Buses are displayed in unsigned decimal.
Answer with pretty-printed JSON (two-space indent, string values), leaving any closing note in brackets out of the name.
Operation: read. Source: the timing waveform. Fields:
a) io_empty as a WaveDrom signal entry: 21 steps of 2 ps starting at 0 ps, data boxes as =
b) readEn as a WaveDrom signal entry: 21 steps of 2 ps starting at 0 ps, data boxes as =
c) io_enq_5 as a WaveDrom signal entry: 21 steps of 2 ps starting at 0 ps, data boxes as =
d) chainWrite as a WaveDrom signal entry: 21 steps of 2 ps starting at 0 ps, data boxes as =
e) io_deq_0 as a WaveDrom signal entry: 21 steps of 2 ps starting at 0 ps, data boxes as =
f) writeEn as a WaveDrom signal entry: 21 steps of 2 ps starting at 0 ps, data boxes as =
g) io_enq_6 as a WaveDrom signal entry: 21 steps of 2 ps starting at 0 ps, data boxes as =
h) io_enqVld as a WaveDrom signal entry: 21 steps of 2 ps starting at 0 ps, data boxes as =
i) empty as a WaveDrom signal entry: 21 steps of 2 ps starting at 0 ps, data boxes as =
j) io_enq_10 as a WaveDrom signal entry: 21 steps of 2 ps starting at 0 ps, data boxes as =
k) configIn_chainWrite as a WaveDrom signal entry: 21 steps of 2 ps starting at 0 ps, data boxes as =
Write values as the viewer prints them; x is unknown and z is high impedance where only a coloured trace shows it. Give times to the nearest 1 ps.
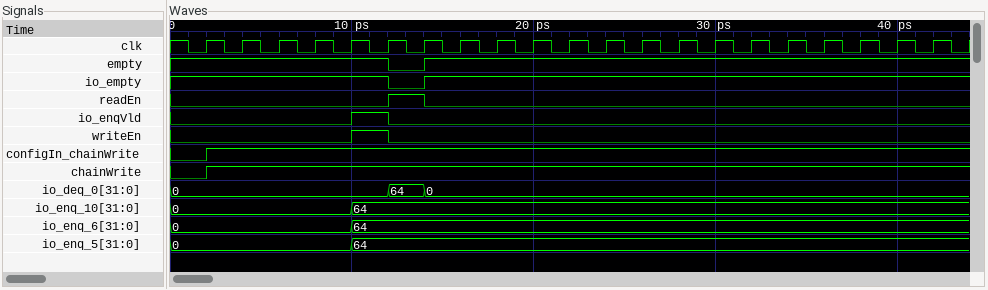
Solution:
{
  "io_empty as a WaveDrom signal entry: 21 steps of 2 ps starting at 0 ps, data boxes as =": "{name: 'io_empty', wave: '1.....01.............'}",
  "readEn as a WaveDrom signal entry: 21 steps of 2 ps starting at 0 ps, data boxes as =": "{name: 'readEn', wave: '0.....10.............'}",
  "io_enq_5 as a WaveDrom signal entry: 21 steps of 2 ps starting at 0 ps, data boxes as =": "{name: 'io_enq_5', wave: '=....=...............', data: '0 64'}",
  "chainWrite as a WaveDrom signal entry: 21 steps of 2 ps starting at 0 ps, data boxes as =": "{name: 'chainWrite', wave: '01...................'}",
  "io_deq_0 as a WaveDrom signal entry: 21 steps of 2 ps starting at 0 ps, data boxes as =": "{name: 'io_deq_0', wave: '=.....==.............', data: '0 64 0'}",
  "writeEn as a WaveDrom signal entry: 21 steps of 2 ps starting at 0 ps, data boxes as =": "{name: 'writeEn', wave: '0....10..............'}",
  "io_enq_6 as a WaveDrom signal entry: 21 steps of 2 ps starting at 0 ps, data boxes as =": "{name: 'io_enq_6', wave: '=....=...............', data: '0 64'}",
  "io_enqVld as a WaveDrom signal entry: 21 steps of 2 ps starting at 0 ps, data boxes as =": "{name: 'io_enqVld', wave: '0....10..............'}",
  "empty as a WaveDrom signal entry: 21 steps of 2 ps starting at 0 ps, data boxes as =": "{name: 'empty', wave: '1.....01.............'}",
  "io_enq_10 as a WaveDrom signal entry: 21 steps of 2 ps starting at 0 ps, data boxes as =": "{name: 'io_enq_10', wave: '=....=...............', data: '0 64'}",
  "configIn_chainWrite as a WaveDrom signal entry: 21 steps of 2 ps starting at 0 ps, data boxes as =": "{name: 'configIn_chainWrite', wave: '01...................'}"
}
